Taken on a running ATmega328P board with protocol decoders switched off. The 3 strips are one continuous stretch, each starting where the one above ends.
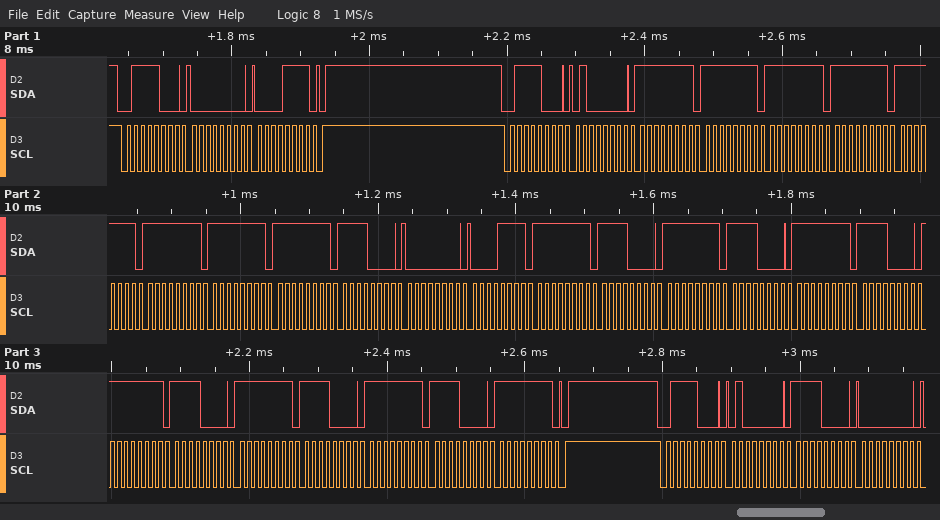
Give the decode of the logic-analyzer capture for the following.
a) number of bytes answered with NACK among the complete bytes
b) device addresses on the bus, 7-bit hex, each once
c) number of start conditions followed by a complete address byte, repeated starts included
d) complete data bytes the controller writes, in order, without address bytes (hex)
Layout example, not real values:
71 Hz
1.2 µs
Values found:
0
0x3C
3
00 0F 40 FF FF FF FF FF FF FF FF F0 00 0F FF F0 FF F0 FF F0 FF F0 FF F0 FF F0 FF 40 F0 00
